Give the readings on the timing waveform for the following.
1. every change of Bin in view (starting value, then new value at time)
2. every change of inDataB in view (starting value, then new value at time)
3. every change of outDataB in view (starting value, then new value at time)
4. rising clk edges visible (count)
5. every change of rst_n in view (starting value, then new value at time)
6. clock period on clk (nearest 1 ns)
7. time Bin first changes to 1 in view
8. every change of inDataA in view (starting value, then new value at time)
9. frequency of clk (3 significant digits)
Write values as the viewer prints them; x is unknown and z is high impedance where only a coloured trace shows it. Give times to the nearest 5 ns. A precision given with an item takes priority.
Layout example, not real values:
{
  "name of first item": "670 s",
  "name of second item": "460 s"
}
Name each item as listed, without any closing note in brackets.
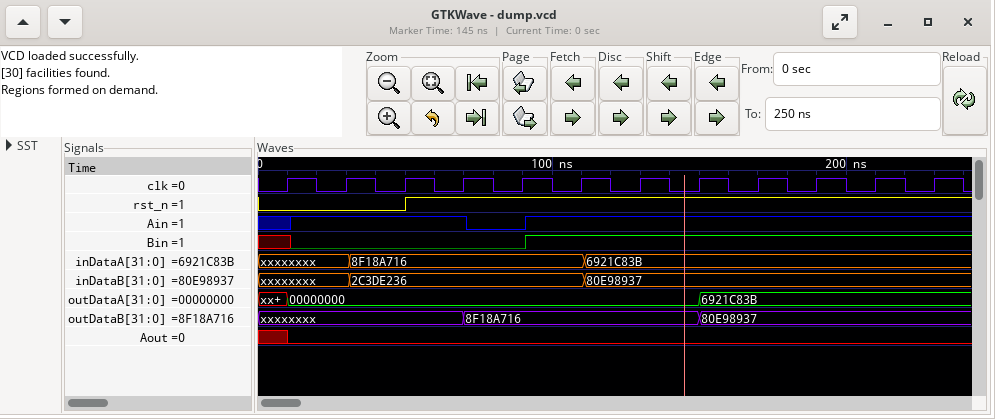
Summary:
{
  "every change of Bin in view": "x, 0 at 10 ns, 1 at 90 ns",
  "every change of inDataB in view": "xxxxxxxx, 2C3DE236 at 30 ns, 80E98937 at 110 ns",
  "every change of outDataB in view": "xxxxxxxx, 8F18A716 at 70 ns, 80E98937 at 150 ns",
  "rising clk edges visible": "12",
  "every change of rst_n in view": "0, 1 at 50 ns",
  "clock period on clk": "20 ns",
  "time Bin first changes to 1 in view": "90 ns",
  "every change of inDataA in view": "xxxxxxxx, 8F18A716 at 30 ns, 6921C83B at 110 ns",
  "frequency of clk": "50.0 MHz"
}
